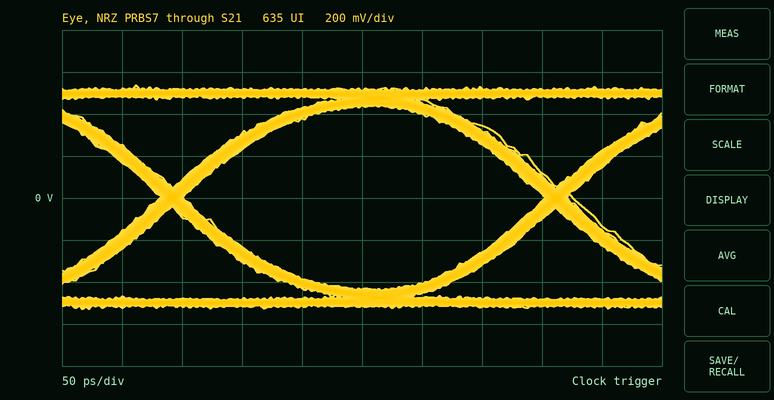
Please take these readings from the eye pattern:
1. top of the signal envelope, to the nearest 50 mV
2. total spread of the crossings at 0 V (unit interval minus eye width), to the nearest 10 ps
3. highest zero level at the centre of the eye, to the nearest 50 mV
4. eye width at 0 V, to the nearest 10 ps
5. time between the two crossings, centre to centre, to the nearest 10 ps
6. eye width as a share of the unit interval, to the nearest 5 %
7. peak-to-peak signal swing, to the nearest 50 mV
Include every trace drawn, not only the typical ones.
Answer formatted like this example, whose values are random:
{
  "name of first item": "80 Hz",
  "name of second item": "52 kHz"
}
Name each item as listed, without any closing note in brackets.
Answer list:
{
  "top of the signal envelope, to the nearest 50 mV": "550 mV",
  "total spread of the crossings at 0 V (unit interval minus eye width), to the nearest 10 ps": "20 ps",
  "highest zero level at the centre of the eye, to the nearest 50 mV": "-450 mV",
  "eye width at 0 V, to the nearest 10 ps": "300 ps",
  "time between the two crossings, centre to centre, to the nearest 10 ps": "320 ps",
  "eye width as a share of the unit interval, to the nearest 5 %": "95 %",
  "peak-to-peak signal swing, to the nearest 50 mV": "1.05 V"
}
